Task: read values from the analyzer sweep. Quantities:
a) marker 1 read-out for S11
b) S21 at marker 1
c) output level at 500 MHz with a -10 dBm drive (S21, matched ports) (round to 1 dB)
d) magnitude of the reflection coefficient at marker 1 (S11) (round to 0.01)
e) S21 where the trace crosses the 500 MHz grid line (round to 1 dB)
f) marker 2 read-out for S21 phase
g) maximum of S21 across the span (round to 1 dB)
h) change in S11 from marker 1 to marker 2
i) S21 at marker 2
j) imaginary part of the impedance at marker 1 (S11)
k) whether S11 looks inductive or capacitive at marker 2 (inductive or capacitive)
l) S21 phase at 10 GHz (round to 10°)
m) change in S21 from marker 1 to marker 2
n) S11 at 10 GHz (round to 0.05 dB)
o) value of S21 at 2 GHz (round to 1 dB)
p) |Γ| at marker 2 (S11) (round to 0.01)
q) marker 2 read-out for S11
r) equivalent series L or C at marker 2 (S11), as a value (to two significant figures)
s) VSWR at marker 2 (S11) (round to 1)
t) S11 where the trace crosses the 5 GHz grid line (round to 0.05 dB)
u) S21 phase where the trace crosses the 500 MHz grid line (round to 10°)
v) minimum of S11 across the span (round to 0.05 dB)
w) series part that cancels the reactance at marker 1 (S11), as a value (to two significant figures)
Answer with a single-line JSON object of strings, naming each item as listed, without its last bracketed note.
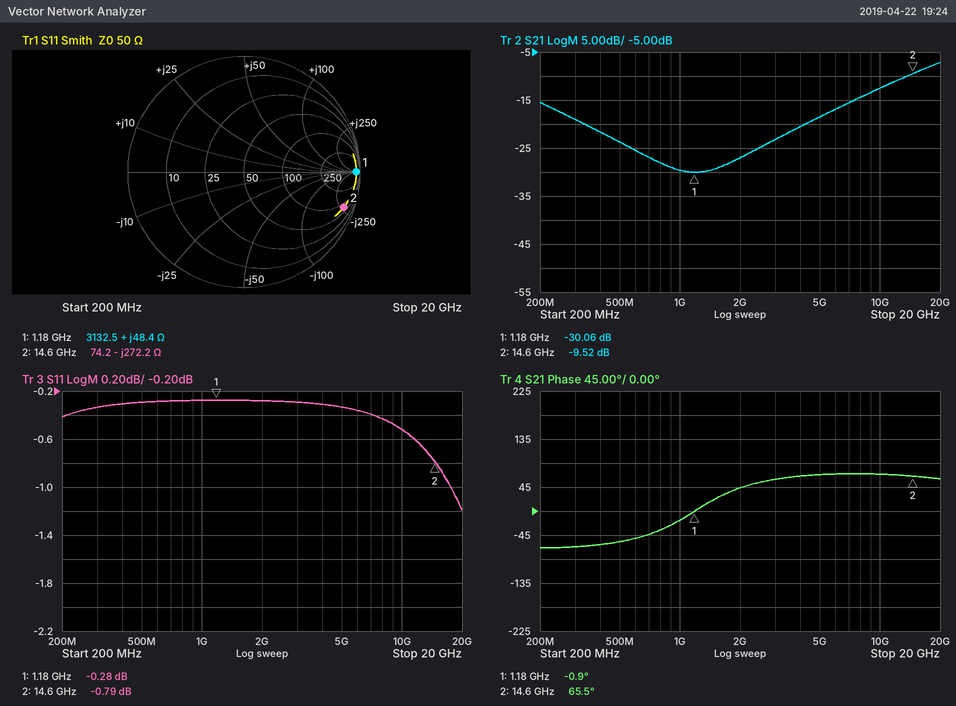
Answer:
{"marker 1 read-out for S11": "-0.28 dB", "S21 at marker 1": "-30.06 dB", "output level at 500 MHz with a -10 dBm drive (S21, matched ports)": "-34 dBm", "magnitude of the reflection coefficient at marker 1 (S11)": "0.97", "S21 where the trace crosses the 500 MHz grid line": "-24 dB", "marker 2 read-out for S21 phase": "65.5°", "maximum of S21 across the span": "-7 dB", "change in S11 from marker 1 to marker 2": "-0.51 dB", "S21 at marker 2": "-9.52 dB", "imaginary part of the impedance at marker 1": "+48.4 Ω", "whether S11 looks inductive or capacitive at marker 2": "capacitive", "S21 phase at 10 GHz": "70°", "change in S21 from marker 1 to marker 2": "20.54 dB", "S11 at 10 GHz": "-0.50 dB", "value of S21 at 2 GHz": "-27 dB", "|Γ| at marker 2 (S11)": "0.91", "marker 2 read-out for S11": "-0.79 dB", "equivalent series L or C at marker 2 (S11), as a value": "40 fF", "VSWR at marker 2 (S11)": "22", "S11 where the trace crosses the 5 GHz grid line": "-0.35 dB", "S21 phase where the trace crosses the 500 MHz grid line": "-60°", "minimum of S11 across the span": "-1.20 dB", "series part that cancels the reactance at marker 1 (S11), as a value": "2.8 pF"}
